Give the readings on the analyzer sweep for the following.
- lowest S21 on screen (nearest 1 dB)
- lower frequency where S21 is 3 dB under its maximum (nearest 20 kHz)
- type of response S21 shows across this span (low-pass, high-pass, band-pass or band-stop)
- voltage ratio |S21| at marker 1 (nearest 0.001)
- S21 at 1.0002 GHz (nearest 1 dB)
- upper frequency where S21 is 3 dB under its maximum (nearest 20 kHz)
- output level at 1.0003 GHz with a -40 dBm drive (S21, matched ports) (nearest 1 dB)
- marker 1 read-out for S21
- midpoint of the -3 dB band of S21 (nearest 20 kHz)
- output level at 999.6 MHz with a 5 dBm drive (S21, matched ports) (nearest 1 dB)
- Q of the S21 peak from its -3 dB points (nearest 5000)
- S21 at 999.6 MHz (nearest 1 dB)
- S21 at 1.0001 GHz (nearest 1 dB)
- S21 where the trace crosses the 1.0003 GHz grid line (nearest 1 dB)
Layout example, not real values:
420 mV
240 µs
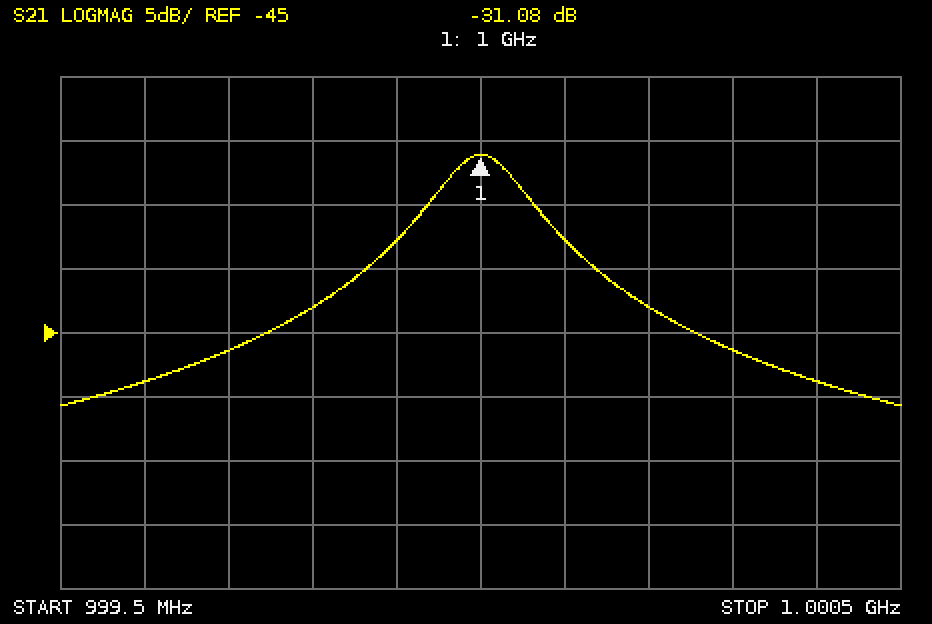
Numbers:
-51 dB
999.94 MHz
band-pass
0.028
-43 dB
1.00006 GHz
-86 dBm
-31.08 dB
1.00000 GHz
-44 dBm
10000
-49 dB
-38 dB
-46 dB
